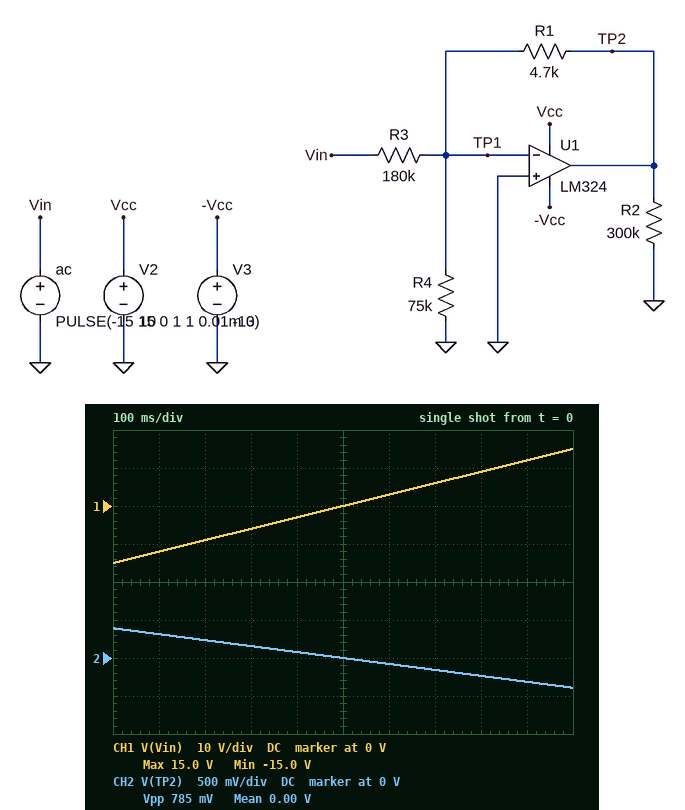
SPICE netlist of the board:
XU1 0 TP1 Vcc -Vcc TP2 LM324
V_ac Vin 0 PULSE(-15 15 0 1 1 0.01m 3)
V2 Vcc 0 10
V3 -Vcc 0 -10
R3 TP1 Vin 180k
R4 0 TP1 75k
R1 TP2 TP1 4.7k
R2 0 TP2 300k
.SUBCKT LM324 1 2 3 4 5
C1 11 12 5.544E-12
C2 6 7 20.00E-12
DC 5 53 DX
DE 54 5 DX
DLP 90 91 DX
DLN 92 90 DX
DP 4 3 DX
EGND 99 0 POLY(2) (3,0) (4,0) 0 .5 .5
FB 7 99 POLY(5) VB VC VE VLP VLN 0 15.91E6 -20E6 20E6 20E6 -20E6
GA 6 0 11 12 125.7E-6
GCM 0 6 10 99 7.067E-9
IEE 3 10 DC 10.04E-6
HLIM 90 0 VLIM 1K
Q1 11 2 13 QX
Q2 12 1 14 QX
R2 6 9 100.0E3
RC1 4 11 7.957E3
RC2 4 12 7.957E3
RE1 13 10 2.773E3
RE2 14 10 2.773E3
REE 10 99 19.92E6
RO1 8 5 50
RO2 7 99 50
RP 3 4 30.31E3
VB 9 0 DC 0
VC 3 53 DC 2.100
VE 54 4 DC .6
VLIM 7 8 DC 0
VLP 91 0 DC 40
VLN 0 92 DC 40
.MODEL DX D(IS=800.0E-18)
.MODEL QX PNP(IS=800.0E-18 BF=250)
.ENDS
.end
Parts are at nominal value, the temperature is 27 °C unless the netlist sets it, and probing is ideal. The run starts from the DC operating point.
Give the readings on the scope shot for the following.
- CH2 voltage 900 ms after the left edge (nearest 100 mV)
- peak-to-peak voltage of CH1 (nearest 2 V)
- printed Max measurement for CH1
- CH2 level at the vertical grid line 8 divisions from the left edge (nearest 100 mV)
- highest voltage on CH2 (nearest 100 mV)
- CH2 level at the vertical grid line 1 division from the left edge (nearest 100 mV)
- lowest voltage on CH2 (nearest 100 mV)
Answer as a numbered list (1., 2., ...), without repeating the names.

1. -300 mV
2. 30 V
3. 15.0 V
4. -200 mV
5. 400 mV
6. 300 mV
7. -400 mV
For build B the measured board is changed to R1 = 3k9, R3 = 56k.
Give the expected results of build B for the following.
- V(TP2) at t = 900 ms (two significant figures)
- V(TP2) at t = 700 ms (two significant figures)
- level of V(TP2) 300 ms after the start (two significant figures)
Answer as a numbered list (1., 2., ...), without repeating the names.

1. -840 mV
2. -420 mV
3. 420 mV
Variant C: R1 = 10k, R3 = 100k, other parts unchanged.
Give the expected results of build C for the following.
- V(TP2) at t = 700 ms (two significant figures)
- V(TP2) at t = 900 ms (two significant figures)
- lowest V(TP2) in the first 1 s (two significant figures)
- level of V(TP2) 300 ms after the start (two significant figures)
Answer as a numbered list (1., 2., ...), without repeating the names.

1. -600 mV
2. -1.2 V
3. -1.5 V
4. 600 mV
